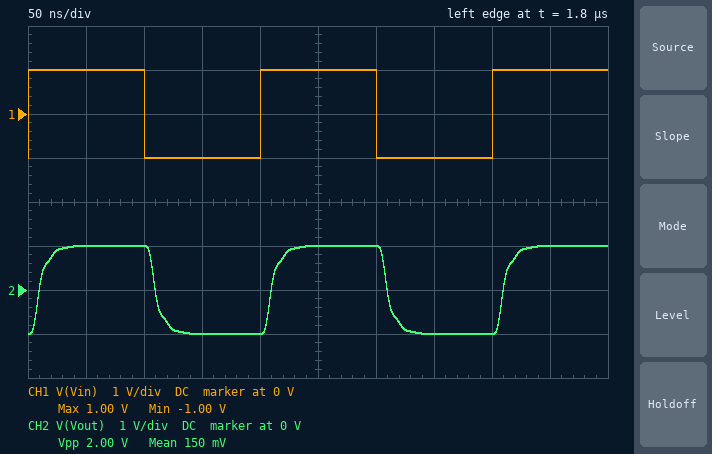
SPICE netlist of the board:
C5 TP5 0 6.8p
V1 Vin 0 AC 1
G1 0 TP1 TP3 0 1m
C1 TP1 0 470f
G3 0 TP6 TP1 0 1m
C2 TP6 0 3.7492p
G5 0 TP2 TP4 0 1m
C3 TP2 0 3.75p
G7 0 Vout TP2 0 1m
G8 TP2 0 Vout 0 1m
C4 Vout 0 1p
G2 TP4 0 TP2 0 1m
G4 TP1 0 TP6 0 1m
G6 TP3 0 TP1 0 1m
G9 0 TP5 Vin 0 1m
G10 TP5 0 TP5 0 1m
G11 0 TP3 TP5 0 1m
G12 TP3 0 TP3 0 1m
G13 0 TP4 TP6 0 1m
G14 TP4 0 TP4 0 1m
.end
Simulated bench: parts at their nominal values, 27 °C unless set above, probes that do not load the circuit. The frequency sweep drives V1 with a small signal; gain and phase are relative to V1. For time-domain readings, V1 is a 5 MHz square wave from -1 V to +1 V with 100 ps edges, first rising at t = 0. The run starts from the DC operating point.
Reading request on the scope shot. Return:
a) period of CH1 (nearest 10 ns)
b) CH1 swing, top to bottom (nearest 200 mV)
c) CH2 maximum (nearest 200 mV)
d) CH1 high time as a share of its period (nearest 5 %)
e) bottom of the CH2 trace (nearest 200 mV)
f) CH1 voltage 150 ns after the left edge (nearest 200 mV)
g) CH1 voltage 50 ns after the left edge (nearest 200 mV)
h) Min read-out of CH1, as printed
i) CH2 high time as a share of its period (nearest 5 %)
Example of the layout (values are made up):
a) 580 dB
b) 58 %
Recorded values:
a) 200 ns
b) 2.0 V
c) 1.0 V
d) 50 %
e) -1.0 V
f) -1.0 V
g) 1.0 V
h) -1.00 V
i) 50 %
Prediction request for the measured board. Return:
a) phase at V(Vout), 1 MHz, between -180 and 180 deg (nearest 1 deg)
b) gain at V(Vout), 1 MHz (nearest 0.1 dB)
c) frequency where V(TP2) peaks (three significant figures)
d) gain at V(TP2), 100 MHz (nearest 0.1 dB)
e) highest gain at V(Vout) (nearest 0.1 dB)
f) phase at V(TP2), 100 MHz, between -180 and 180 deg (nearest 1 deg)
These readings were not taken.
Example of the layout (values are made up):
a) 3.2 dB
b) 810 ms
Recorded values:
a) -4 deg
b) 0 dB
c) 71.5 MHz
d) -22.4 dB
e) 0 dB
f) 163 deg
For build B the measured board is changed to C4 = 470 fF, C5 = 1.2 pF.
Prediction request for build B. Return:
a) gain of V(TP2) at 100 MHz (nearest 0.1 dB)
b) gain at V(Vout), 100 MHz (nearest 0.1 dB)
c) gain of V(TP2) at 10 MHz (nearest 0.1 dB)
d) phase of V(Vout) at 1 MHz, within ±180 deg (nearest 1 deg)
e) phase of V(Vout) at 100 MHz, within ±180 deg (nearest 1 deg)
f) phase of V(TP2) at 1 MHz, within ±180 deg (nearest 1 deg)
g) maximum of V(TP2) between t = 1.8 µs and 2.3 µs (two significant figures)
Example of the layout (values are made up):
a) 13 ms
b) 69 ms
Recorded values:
a) -12.6 dB
b) -2.0 dB
c) -30.7 dB
d) -2 deg
e) -164 deg
f) 88 deg
g) 220 mV
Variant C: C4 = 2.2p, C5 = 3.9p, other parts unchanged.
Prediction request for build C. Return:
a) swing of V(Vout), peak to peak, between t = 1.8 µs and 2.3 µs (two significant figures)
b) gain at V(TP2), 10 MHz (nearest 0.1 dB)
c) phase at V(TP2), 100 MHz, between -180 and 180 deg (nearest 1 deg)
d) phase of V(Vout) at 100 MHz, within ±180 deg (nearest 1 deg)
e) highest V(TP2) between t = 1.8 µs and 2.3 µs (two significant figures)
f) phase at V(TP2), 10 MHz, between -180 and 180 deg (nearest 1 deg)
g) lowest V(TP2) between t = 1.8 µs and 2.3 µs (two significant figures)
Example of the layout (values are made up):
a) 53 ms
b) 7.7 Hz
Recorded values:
a) 2.1 V
b) -17.4 dB
c) 151 deg
d) 61 deg
e) 480 mV
f) 55 deg
g) -480 mV
